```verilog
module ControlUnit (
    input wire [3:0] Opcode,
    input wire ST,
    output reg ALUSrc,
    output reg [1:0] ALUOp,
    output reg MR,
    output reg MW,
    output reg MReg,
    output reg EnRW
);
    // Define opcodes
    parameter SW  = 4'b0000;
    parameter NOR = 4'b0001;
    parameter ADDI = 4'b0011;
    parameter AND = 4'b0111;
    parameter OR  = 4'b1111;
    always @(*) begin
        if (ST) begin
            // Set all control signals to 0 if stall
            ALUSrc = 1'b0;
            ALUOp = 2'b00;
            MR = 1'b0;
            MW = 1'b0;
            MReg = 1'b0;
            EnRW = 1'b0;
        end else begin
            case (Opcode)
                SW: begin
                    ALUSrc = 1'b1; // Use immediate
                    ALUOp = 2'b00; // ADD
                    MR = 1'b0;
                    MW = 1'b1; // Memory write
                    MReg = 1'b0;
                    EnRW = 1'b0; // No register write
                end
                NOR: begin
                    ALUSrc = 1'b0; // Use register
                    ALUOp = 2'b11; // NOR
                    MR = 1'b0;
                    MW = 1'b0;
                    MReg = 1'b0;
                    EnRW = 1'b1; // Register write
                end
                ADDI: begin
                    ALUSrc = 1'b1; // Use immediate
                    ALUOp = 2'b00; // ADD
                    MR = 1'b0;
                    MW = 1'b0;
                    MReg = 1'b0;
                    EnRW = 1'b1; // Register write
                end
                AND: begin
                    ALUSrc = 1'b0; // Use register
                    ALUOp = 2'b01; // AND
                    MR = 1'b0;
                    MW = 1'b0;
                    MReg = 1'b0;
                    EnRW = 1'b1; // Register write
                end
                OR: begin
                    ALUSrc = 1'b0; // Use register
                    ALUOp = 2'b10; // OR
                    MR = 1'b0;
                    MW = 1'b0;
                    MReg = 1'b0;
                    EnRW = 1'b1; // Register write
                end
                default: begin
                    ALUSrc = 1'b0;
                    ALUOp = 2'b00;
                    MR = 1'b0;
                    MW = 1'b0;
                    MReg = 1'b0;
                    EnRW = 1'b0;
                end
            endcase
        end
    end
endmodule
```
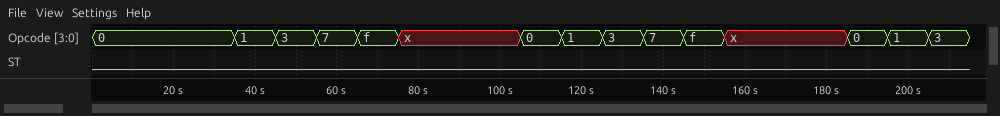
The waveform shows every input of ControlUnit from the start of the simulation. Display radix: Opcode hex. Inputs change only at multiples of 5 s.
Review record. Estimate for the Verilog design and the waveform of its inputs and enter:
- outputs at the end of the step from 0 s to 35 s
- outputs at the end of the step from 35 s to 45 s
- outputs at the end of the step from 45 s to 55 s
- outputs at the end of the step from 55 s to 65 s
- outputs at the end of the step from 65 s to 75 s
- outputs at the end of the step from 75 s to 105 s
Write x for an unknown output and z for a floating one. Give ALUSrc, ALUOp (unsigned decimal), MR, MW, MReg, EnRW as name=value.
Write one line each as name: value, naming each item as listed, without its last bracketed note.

outputs at the end of the step from 0 s to 35 s: ALUSrc=1, ALUOp=0, MR=0, MW=1, MReg=0, EnRW=0
outputs at the end of the step from 35 s to 45 s: ALUSrc=0, ALUOp=3, MR=0, MW=0, MReg=0, EnRW=1
outputs at the end of the step from 45 s to 55 s: ALUSrc=1, ALUOp=0, MR=0, MW=0, MReg=0, EnRW=1
outputs at the end of the step from 55 s to 65 s: ALUSrc=0, ALUOp=1, MR=0, MW=0, MReg=0, EnRW=1
outputs at the end of the step from 65 s to 75 s: ALUSrc=0, ALUOp=2, MR=0, MW=0, MReg=0, EnRW=1
outputs at the end of the step from 75 s to 105 s: ALUSrc=0, ALUOp=0, MR=0, MW=0, MReg=0, EnRW=0
